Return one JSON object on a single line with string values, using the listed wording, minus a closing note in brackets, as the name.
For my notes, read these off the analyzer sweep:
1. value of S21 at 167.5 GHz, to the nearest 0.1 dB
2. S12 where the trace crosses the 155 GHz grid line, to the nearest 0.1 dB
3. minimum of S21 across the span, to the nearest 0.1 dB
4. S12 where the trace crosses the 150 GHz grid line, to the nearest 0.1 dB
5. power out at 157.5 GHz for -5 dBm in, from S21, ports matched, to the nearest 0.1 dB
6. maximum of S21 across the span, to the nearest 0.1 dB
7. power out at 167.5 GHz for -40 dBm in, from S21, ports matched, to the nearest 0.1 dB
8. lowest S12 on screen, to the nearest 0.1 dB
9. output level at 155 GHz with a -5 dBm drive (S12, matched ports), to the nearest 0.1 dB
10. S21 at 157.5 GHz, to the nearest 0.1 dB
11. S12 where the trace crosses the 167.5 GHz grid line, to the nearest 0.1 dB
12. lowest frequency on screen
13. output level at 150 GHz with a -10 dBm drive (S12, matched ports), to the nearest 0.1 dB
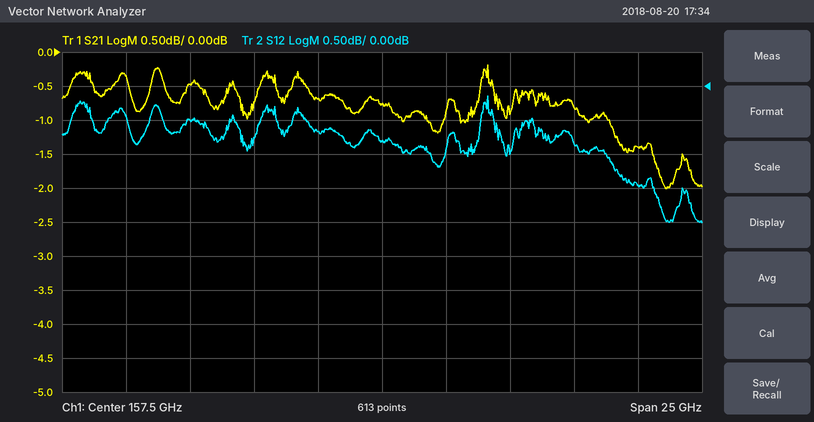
{"value of S21 at 167.5 GHz, to the nearest 0.1 dB": "-1.4 dB", "S12 where the trace crosses the 155 GHz grid line, to the nearest 0.1 dB": "-0.7 dB", "minimum of S21 across the span, to the nearest 0.1 dB": "-2.0 dB", "S12 where the trace crosses the 150 GHz grid line, to the nearest 0.1 dB": "-0.5 dB", "power out at 157.5 GHz for -5 dBm in, from S21, ports matched, to the nearest 0.1 dB": "-5.8 dBm", "maximum of S21 across the span, to the nearest 0.1 dB": "-0.2 dB", "power out at 167.5 GHz for -40 dBm in, from S21, ports matched, to the nearest 0.1 dB": "-41.4 dBm", "lowest S12 on screen, to the nearest 0.1 dB": "-2.0 dB", "output level at 155 GHz with a -5 dBm drive (S12, matched ports), to the nearest 0.1 dB": "-5.7 dBm", "S21 at 157.5 GHz, to the nearest 0.1 dB": "-0.8 dB", "S12 where the trace crosses the 167.5 GHz grid line, to the nearest 0.1 dB": "-1.5 dB", "lowest frequency on screen": "145 GHz", "output level at 150 GHz with a -10 dBm drive (S12, matched ports), to the nearest 0.1 dB": "-10.5 dBm"}
